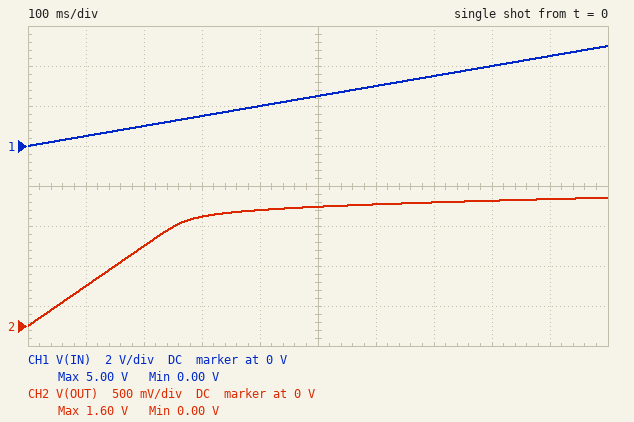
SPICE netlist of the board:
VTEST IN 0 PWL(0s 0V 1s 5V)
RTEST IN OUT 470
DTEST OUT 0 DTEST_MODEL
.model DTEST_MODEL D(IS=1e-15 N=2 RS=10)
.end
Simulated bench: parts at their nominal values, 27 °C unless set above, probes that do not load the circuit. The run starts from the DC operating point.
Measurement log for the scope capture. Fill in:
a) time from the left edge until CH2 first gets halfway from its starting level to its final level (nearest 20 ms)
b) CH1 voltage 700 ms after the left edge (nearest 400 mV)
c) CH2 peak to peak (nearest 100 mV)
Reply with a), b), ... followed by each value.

a) 160 ms
b) 3.6 V
c) 1.6 V
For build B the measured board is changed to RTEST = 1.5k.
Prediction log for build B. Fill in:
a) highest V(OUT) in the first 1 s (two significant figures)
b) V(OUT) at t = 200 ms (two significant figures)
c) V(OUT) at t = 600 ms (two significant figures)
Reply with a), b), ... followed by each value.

a) 1.5 V
b) 1.0 V
c) 1.4 V
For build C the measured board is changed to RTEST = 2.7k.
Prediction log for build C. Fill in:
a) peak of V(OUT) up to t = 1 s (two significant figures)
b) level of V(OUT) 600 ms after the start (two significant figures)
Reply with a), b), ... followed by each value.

a) 1.5 V
b) 1.4 V
